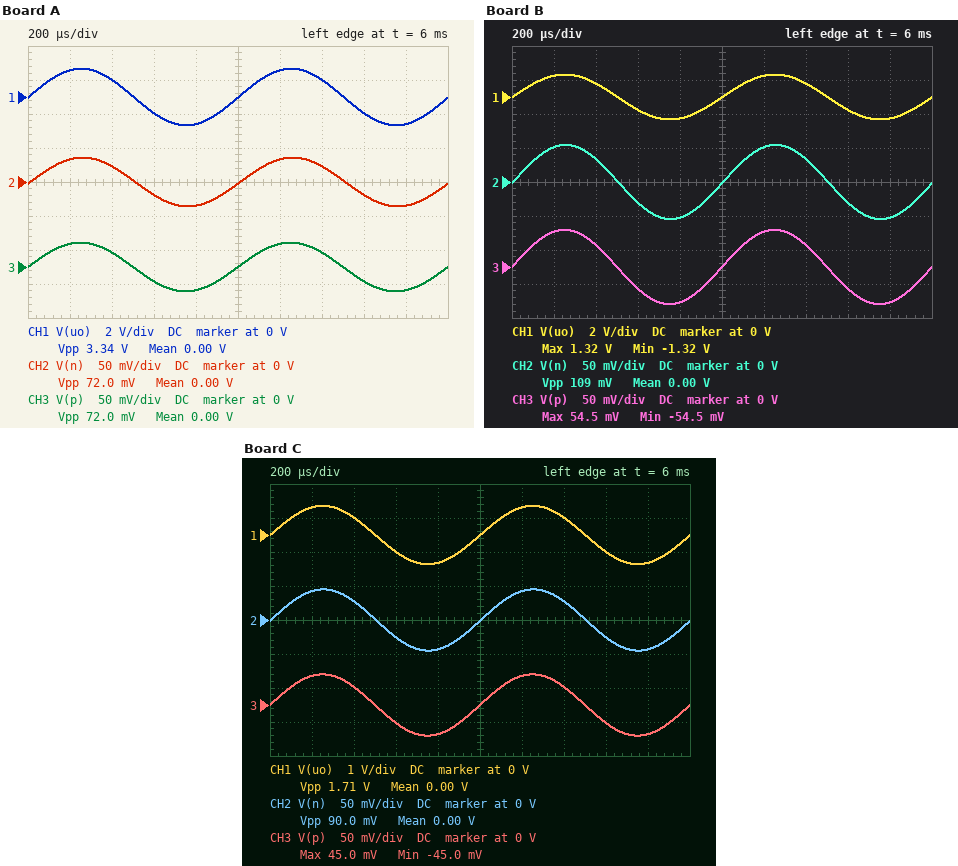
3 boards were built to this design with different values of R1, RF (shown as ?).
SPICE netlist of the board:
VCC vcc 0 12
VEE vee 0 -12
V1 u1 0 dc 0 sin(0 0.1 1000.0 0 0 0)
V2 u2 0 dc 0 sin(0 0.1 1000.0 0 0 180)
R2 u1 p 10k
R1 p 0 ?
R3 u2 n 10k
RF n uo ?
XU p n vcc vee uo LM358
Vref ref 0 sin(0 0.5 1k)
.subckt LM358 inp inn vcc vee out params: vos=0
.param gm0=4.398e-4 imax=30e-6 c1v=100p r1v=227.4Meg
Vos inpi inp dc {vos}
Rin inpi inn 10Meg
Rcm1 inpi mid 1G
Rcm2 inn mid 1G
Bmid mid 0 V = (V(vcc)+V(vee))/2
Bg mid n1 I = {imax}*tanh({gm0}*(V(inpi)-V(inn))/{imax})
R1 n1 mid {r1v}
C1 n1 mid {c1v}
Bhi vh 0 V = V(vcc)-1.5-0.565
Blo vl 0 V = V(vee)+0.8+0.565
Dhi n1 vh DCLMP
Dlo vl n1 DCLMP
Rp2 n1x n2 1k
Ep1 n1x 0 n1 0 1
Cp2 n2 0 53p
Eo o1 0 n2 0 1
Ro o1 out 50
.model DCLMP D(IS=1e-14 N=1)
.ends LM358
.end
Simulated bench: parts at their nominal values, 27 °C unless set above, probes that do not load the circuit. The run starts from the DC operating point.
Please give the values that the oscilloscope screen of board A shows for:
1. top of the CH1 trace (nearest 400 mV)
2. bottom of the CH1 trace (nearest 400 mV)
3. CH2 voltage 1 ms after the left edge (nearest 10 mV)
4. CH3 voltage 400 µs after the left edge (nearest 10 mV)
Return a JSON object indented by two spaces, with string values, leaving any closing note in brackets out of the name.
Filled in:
{
  "top of the CH1 trace": "1.6 V",
  "bottom of the CH1 trace": "-1.6 V",
  "CH2 voltage 1 ms after the left edge": "0 V",
  "CH3 voltage 400 µs after the left edge": "20 mV"
}
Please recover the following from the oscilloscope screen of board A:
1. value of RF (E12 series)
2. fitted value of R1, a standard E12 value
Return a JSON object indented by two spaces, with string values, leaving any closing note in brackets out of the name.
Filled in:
{
  "value of RF": "120 kΩ",
  "fitted value of R1, a standard E12 value": "5.6 kΩ"
}
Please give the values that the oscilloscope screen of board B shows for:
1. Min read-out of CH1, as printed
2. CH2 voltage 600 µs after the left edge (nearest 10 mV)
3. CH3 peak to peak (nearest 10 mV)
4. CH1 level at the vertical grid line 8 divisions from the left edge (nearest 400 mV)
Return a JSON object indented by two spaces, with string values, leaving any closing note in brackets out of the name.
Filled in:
{
  "Min read-out of CH1, as printed": "-1.32 V",
  "CH2 voltage 600 µs after the left edge": "-30 mV",
  "CH3 peak to peak": "110 mV",
  "CH1 level at the vertical grid line 8 divisions from the left edge": "-800 mV"
}
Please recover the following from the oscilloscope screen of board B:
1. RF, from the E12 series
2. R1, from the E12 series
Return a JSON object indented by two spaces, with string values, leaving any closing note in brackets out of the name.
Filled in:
{
  "RF, from the E12 series": "82 kΩ",
  "R1, from the E12 series": "12 kΩ"
}
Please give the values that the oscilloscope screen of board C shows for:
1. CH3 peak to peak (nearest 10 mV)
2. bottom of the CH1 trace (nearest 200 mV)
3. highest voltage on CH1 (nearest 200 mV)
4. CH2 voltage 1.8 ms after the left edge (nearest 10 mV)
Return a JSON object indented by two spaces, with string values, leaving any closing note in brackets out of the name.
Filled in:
{
  "CH3 peak to peak": "90 mV",
  "bottom of the CH1 trace": "-800 mV",
  "highest voltage on CH1": "800 mV",
  "CH2 voltage 1.8 ms after the left edge": "-40 mV"
}
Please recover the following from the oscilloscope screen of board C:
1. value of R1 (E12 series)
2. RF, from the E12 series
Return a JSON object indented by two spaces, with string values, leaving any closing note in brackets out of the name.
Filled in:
{
  "value of R1": "8.2 kΩ",
  "RF, from the E12 series": "56 kΩ"
}
